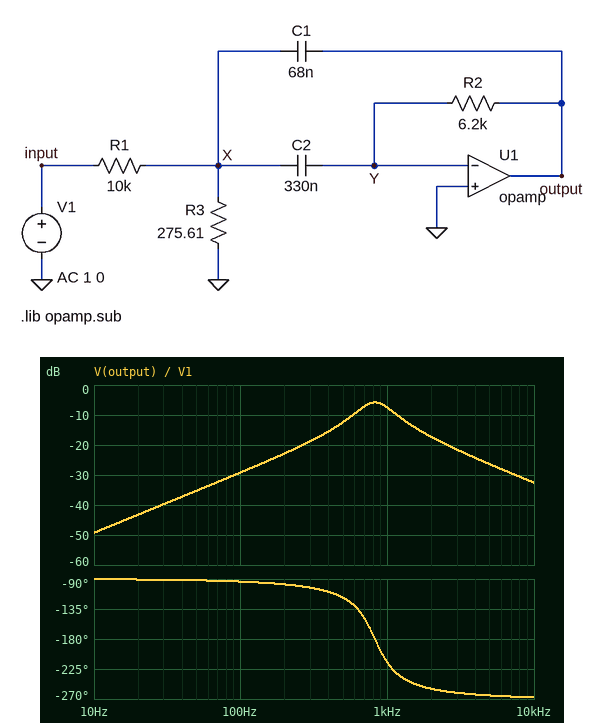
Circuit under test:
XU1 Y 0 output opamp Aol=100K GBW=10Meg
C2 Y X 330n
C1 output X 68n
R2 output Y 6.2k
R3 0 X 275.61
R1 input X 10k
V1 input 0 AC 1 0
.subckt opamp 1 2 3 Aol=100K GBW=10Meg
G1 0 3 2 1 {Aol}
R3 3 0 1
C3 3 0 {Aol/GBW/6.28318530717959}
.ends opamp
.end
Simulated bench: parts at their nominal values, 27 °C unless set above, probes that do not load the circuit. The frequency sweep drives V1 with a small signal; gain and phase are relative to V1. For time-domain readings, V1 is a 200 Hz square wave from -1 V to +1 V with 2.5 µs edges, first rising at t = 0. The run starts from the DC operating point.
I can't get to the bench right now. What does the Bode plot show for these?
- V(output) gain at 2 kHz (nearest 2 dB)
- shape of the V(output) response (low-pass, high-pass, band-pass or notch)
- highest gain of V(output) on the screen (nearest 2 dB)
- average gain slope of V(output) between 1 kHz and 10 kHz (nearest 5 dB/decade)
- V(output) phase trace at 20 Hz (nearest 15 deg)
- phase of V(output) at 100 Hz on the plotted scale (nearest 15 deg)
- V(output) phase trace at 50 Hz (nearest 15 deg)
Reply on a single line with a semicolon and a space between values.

-18 dB; band-pass; -6 dB; -25 dB/decade; -90 deg; -90 deg; -90 deg
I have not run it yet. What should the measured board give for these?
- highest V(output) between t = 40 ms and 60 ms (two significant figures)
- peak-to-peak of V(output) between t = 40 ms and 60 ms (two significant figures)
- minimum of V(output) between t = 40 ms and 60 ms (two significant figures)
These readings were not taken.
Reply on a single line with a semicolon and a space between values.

380 mV; 760 mV; -380 mV
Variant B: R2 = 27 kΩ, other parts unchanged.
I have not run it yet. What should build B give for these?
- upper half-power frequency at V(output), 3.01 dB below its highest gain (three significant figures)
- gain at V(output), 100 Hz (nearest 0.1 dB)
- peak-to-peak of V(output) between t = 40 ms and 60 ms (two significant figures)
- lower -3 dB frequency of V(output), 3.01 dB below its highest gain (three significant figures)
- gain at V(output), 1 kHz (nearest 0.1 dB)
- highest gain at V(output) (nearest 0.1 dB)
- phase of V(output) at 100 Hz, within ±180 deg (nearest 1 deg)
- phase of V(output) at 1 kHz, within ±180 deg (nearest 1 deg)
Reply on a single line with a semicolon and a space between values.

450 Hz; -15.9 dB; 1.4 V; 346 Hz; -11.2 dB; 7.0 dB; -94 deg; 97 deg
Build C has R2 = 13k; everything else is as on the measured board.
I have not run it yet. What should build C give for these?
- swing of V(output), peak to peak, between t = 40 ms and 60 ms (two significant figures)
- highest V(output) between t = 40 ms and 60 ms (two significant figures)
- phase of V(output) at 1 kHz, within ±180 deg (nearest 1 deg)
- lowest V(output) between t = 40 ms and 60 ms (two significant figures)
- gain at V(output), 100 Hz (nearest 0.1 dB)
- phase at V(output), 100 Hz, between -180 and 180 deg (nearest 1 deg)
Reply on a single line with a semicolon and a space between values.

1.4 V; 710 mV; 108 deg; -710 mV; -22.6 dB; -94 deg
